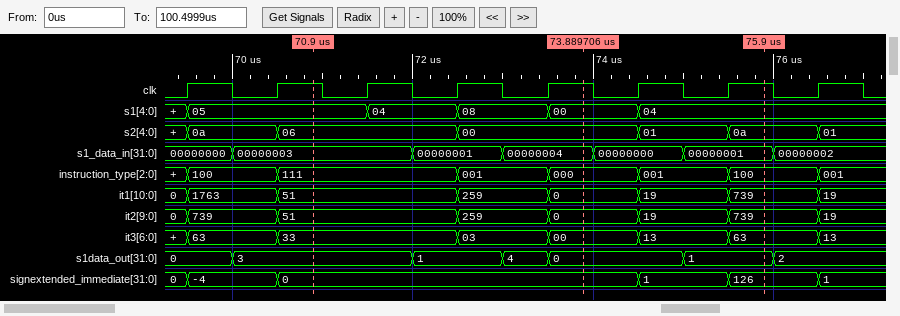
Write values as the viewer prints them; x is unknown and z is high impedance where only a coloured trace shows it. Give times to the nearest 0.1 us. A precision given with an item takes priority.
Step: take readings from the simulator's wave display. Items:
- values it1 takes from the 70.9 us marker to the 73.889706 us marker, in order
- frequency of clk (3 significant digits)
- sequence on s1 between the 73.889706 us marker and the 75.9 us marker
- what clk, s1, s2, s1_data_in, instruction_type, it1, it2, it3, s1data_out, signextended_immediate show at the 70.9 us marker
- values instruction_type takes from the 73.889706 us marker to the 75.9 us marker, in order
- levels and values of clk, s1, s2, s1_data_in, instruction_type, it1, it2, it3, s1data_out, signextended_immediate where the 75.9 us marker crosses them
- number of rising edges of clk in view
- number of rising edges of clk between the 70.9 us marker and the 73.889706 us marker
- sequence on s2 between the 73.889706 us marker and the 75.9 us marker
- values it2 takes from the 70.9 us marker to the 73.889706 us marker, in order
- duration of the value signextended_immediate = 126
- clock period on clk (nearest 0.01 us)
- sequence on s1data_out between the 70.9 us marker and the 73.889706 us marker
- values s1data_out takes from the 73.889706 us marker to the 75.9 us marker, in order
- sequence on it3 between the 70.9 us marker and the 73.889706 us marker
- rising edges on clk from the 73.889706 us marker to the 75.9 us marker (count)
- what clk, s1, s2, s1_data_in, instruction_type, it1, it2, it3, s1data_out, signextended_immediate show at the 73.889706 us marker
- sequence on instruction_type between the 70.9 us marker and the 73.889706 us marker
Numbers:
51, 259, 0
1.00 MHz
00, 04
clk=1, s1=05, s2=06, s1_data_in=00000003, instruction_type=111, it1=51, it2=51, it3=33, s1data_out=3, signextended_immediate=0
000, 001, 100
clk=1, s1=04, s2=0a, s1_data_in=00000001, instruction_type=100, it1=739, it2=739, it3=63, s1data_out=1, signextended_immediate=126
8
3
00, 01, 0a
51, 259, 0
1 us
1 us
3, 1, 4, 0
0, 1
33, 03, 00
2
clk=1, s1=00, s2=00, s1_data_in=00000004, instruction_type=000, it1=0, it2=0, it3=00, s1data_out=0, signextended_immediate=0
111, 001, 000
